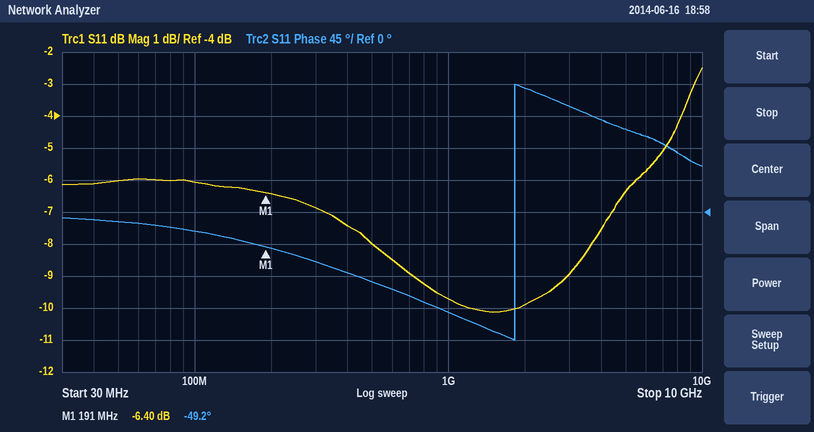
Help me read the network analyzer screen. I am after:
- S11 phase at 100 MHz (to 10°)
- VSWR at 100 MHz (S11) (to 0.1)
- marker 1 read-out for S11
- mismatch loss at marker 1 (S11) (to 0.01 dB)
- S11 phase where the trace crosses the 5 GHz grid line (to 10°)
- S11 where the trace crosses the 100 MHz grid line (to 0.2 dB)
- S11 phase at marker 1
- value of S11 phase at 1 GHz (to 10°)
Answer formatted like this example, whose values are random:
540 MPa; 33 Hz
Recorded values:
-30°; 3.0; -6.40 dB; 1.13 dB; 120°; -6.0 dB; -49.2°; -140°
